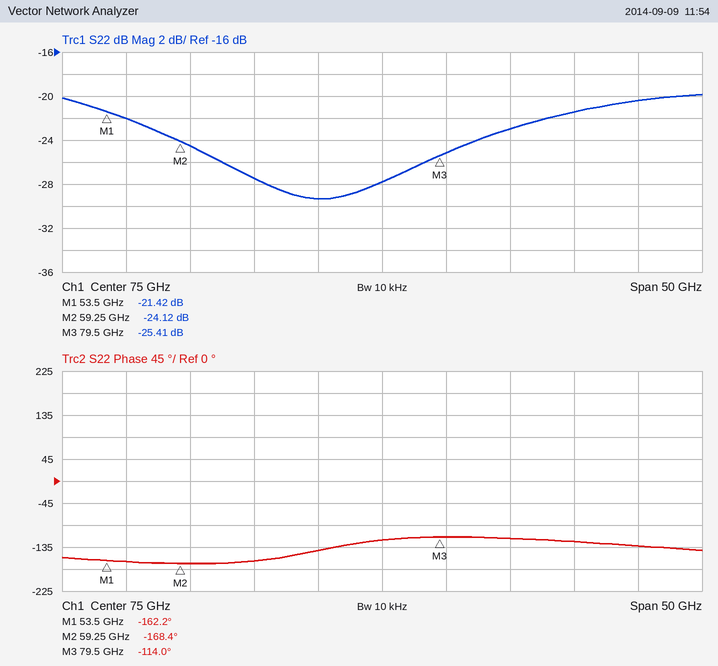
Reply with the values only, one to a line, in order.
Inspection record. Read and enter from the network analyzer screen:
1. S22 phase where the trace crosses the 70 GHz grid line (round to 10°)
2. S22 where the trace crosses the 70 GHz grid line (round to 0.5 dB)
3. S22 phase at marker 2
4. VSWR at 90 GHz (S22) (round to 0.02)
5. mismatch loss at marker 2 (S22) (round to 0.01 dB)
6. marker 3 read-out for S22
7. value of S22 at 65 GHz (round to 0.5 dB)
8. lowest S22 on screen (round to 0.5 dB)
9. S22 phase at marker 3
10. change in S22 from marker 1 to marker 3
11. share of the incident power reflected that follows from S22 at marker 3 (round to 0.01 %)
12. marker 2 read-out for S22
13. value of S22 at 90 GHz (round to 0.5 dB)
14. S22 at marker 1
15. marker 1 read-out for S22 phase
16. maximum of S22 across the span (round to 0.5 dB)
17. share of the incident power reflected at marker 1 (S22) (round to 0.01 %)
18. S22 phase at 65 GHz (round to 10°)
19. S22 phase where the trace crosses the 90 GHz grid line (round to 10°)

-140°
-29.5 dB
-168.4°
1.18
0.02 dB
-25.41 dB
-27.5 dB
-29.5 dB
-114.0°
-3.99 dB
0.29 %
-24.12 dB
-21.5 dB
-21.42 dB
-162.2°
-20.0 dB
0.72 %
-160°
-120°
